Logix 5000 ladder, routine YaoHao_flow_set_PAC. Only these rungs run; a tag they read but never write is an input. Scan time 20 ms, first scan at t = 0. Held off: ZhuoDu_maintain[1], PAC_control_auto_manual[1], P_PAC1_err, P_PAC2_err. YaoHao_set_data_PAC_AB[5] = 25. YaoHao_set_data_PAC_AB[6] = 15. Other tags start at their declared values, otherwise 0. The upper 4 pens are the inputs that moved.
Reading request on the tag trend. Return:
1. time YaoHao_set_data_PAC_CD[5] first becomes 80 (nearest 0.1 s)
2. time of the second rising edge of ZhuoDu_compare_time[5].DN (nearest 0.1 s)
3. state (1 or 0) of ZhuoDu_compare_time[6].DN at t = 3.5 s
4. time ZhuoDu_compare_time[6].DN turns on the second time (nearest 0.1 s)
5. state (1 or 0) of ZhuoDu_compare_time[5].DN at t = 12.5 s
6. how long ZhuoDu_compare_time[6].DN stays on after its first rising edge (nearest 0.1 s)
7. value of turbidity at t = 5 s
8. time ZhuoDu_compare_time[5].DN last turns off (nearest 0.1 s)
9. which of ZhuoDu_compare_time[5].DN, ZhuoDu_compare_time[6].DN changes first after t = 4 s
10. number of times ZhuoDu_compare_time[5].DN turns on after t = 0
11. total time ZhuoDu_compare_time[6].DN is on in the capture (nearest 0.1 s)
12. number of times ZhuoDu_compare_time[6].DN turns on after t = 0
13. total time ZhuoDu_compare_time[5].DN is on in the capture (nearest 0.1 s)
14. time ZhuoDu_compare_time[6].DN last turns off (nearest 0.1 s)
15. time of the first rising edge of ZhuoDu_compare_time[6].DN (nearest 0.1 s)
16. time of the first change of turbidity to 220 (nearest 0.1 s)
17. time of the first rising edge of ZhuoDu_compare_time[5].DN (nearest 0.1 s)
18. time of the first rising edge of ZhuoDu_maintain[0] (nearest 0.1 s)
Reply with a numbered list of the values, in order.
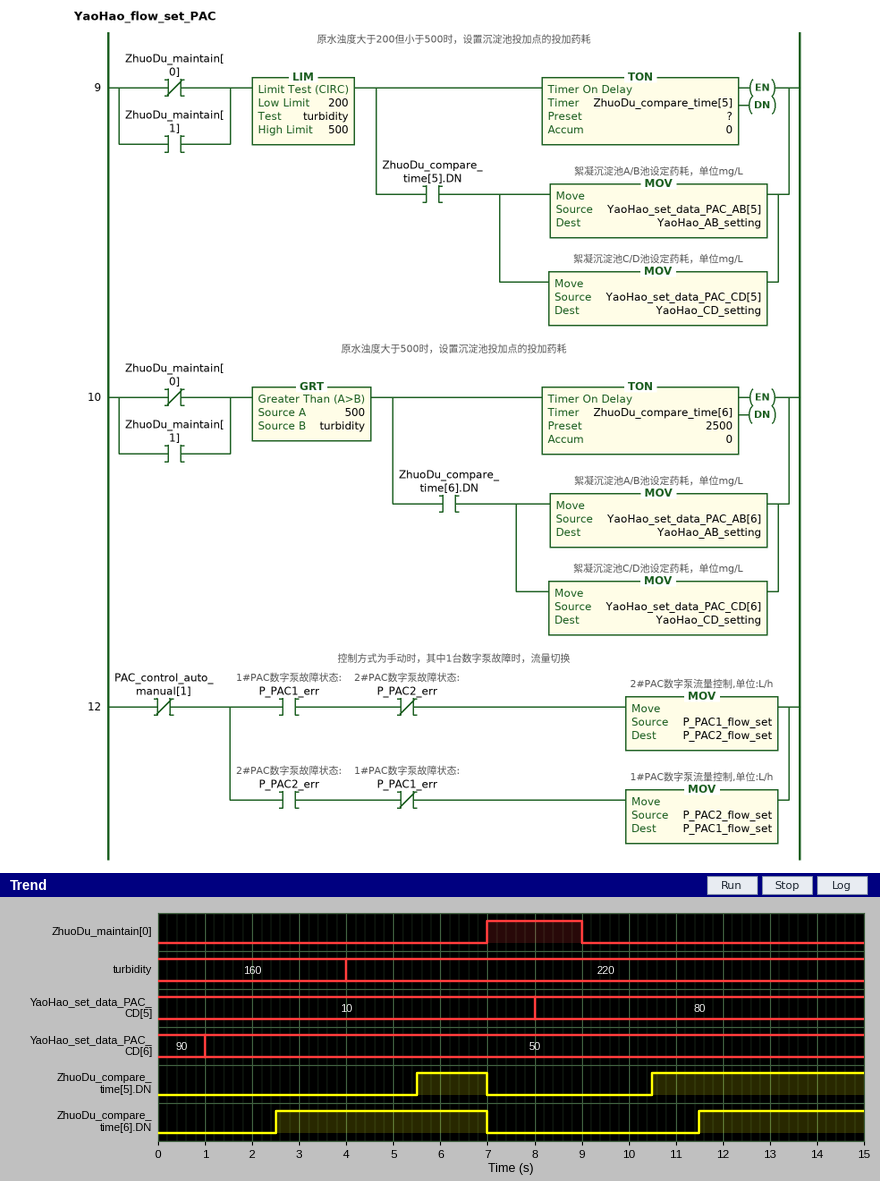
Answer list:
1. 8.0 s
2. 10.5 s
3. 1
4. 11.5 s
5. 1
6. 4.5 s
7. 220
8. 7.0 s
9. ZhuoDu_compare_time[5].DN
10. 2
11. 8.0 s
12. 2
13. 6.0 s
14. 7.0 s
15. 2.5 s
16. 4.0 s
17. 5.5 s
18. 7.0 s
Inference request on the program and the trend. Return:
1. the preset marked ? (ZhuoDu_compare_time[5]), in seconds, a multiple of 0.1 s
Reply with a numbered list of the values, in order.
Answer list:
1. 1.5 s
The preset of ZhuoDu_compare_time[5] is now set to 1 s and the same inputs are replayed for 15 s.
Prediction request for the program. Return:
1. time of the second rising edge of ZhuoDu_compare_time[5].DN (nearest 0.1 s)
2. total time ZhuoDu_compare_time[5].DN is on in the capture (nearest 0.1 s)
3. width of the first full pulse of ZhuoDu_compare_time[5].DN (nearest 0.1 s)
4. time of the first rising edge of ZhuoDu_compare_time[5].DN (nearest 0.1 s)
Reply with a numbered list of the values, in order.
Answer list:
1. 10.0 s
2. 7.0 s
3. 2.0 s
4. 5.0 s
